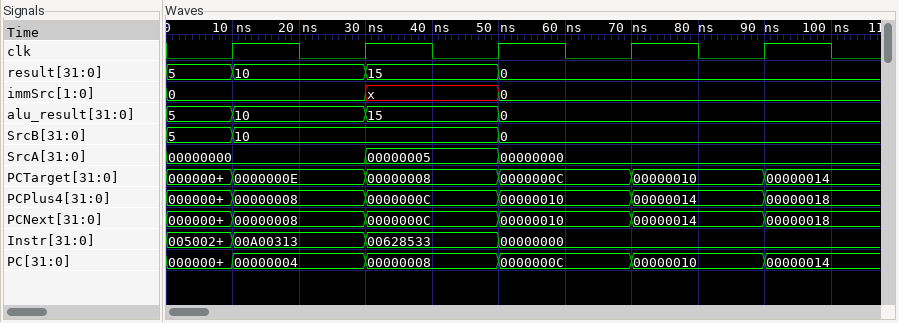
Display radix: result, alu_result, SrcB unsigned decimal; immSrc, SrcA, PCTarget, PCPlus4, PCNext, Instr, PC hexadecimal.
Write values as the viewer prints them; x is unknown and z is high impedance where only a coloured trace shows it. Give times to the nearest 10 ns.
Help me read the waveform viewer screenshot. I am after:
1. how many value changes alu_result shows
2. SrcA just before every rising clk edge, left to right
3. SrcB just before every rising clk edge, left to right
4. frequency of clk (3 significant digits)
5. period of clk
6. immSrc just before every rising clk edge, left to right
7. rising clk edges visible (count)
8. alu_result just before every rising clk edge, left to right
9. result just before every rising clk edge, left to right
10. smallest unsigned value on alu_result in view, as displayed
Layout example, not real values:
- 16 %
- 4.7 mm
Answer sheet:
- 3
- 00000000, 00000000, 00000005, 00000000, 00000000
- 5, 10, 10, 0, 0
- 50.0 MHz
- 20 ns
- 0, 0, x, 0, 0
- 5
- 5, 10, 15, 0, 0
- 5, 10, 15, 0, 0
- 0
